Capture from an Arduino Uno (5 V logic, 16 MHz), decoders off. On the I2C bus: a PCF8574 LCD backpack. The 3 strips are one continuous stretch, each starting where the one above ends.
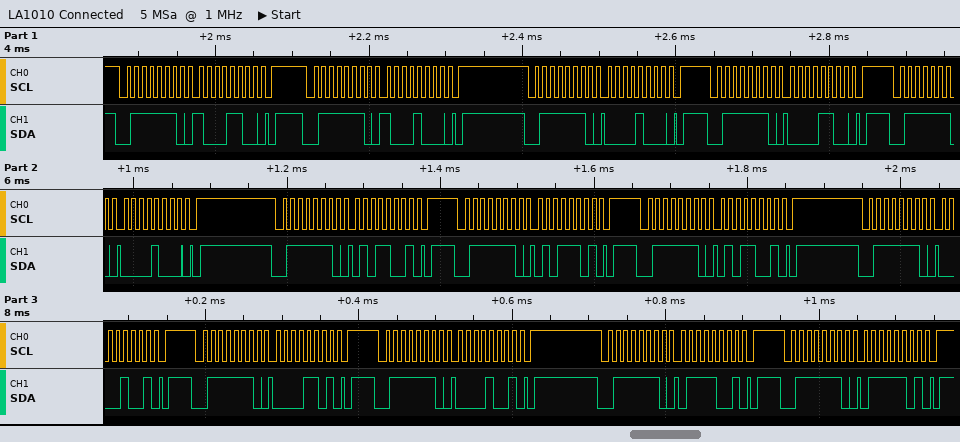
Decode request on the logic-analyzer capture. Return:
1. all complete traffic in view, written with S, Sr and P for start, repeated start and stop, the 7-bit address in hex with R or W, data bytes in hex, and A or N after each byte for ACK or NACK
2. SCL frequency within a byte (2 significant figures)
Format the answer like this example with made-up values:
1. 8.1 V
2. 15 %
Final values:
1. S 3FW A 8C A P S 3FW A 88 A P S 3FW A 08 A P S 3FW A 0C A P S 3FW A 08 A P S 3FW A 59 A P S 3FW A 5D A P S 3FW A 59 A P S 3FW A 09 A P S 3FW A 0D A P S 3FW A 09 A P S 3FW A 79 A P S 3FW A 7D A P
2. 100 kHz
